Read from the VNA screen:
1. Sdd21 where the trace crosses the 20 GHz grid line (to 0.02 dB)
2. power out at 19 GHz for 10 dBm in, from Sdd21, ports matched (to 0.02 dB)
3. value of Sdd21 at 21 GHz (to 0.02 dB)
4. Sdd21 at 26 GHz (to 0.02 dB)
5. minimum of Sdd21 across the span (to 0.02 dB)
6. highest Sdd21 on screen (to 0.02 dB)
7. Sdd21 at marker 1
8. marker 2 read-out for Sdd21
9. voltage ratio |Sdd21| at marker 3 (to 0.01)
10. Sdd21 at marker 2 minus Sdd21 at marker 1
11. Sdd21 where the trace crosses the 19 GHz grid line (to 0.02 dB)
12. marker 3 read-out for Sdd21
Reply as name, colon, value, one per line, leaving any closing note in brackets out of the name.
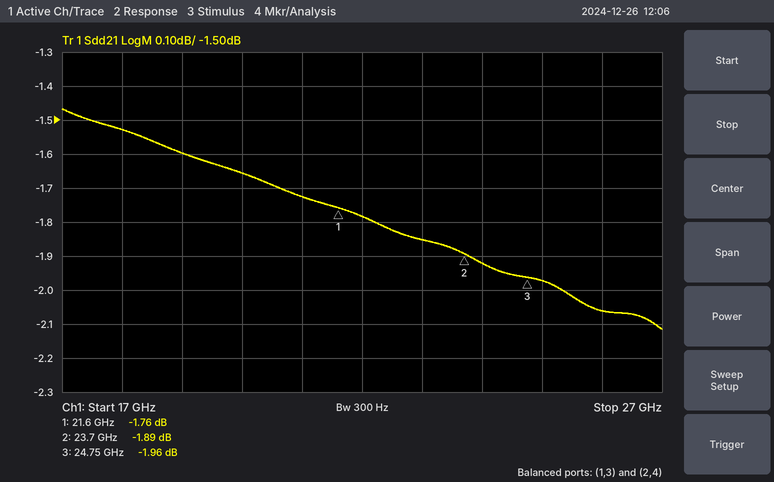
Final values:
Sdd21 where the trace crosses the 20 GHz grid line: -1.66 dB
power out at 19 GHz for 10 dBm in, from Sdd21, ports matched: 8.40 dBm
value of Sdd21 at 21 GHz: -1.72 dB
Sdd21 at 26 GHz: -2.06 dB
minimum of Sdd21 across the span: -2.12 dB
highest Sdd21 on screen: -1.46 dB
Sdd21 at marker 1: -1.76 dB
marker 2 read-out for Sdd21: -1.89 dB
voltage ratio |Sdd21| at marker 3: 0.80
Sdd21 at marker 2 minus Sdd21 at marker 1: -0.13 dB
Sdd21 where the trace crosses the 19 GHz grid line: -1.60 dB
marker 3 read-out for Sdd21: -1.96 dB
